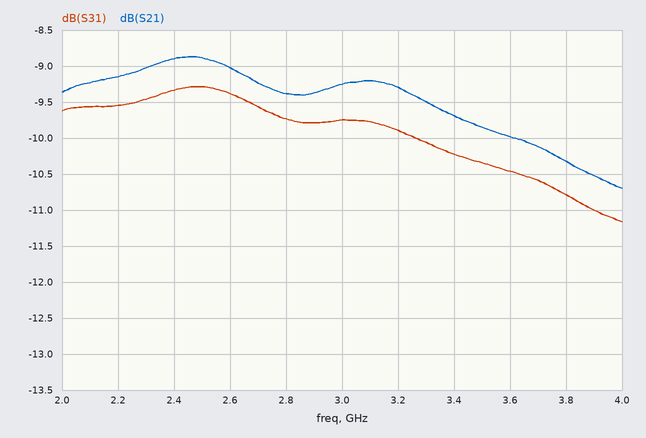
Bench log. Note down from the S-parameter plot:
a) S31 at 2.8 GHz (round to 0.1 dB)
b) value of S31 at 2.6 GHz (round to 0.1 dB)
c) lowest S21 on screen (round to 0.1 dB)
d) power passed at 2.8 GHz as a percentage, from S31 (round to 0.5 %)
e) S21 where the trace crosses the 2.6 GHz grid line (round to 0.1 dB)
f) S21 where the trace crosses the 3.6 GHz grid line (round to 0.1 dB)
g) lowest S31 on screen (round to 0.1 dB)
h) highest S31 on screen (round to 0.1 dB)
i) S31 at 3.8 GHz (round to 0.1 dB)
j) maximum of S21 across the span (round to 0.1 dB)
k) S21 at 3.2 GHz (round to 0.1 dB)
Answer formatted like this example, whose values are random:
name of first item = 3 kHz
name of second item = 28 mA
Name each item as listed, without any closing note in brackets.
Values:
S31 at 2.8 GHz = -9.7 dB
value of S31 at 2.6 GHz = -9.4 dB
lowest S21 on screen = -10.7 dB
power passed at 2.8 GHz as a percentage, from S31 = 10.5 %
S21 where the trace crosses the 2.6 GHz grid line = -9.0 dB
S21 where the trace crosses the 3.6 GHz grid line = -10.0 dB
lowest S31 on screen = -11.2 dB
highest S31 on screen = -9.3 dB
S31 at 3.8 GHz = -10.8 dB
maximum of S21 across the span = -8.9 dB
S21 at 3.2 GHz = -9.3 dB
